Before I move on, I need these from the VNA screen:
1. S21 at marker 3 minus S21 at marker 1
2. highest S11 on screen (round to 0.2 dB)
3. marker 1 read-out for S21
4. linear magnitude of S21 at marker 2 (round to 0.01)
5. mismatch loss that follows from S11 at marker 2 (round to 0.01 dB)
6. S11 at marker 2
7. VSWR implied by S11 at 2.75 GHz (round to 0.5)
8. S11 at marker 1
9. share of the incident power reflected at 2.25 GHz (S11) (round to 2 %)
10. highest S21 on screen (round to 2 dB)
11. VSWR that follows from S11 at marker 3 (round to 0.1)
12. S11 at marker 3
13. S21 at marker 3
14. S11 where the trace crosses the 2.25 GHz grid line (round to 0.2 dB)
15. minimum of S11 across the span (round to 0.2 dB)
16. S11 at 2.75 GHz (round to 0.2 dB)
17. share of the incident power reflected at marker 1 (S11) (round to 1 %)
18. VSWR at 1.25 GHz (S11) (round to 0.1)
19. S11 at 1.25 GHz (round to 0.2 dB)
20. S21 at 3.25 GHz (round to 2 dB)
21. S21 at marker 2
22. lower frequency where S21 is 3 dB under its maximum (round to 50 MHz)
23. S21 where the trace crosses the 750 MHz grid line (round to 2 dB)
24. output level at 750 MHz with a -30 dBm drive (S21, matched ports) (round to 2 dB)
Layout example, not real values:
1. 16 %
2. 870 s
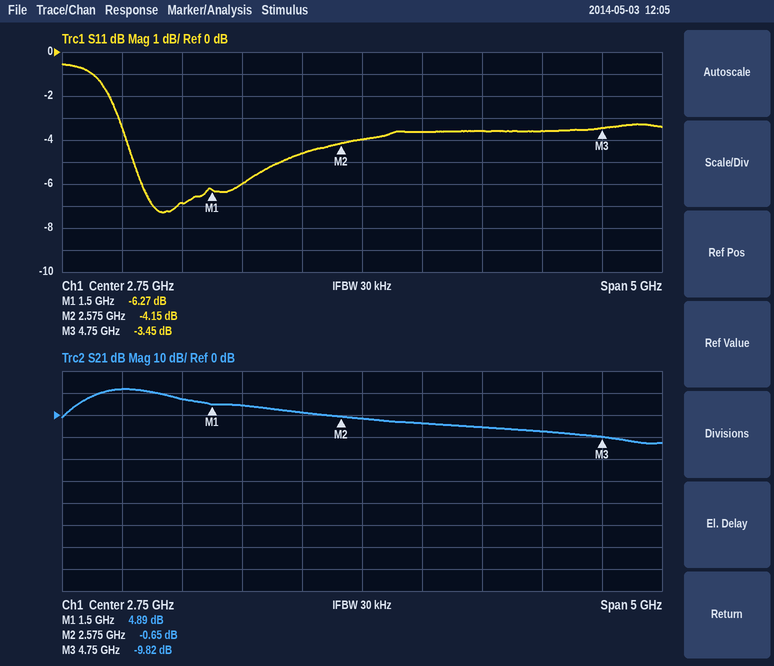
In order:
1. -14.71 dB
2. -0.6 dB
3. 4.89 dB
4. 0.93
5. 2.11 dB
6. -4.15 dB
7. 4.5
8. -6.27 dB
9. 34 %
10. 12 dB
11. 5.1
12. -3.45 dB
13. -9.82 dB
14. -4.6 dB
15. -7.2 dB
16. -4.0 dB
17. 24 %
18. 2.7
19. -6.8 dB
20. -4 dB
21. -0.65 dB
22. 500 MHz
23. 12 dB
24. -18 dBm
